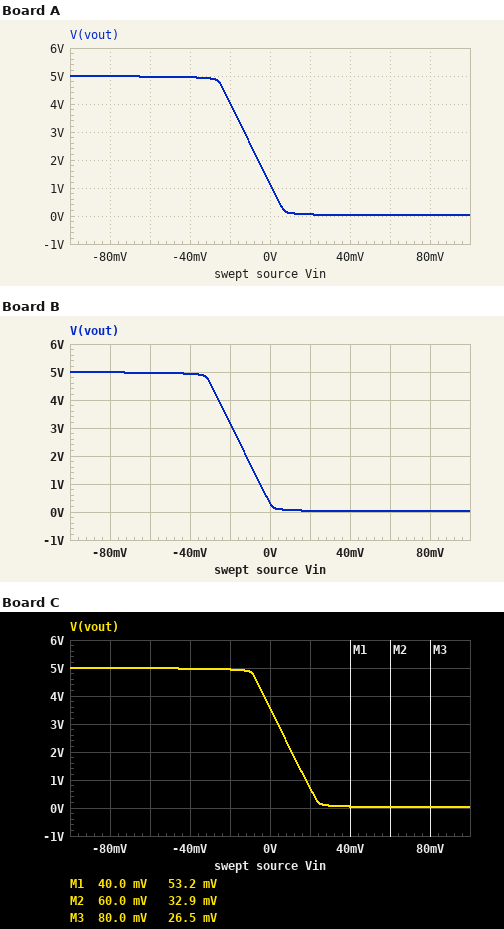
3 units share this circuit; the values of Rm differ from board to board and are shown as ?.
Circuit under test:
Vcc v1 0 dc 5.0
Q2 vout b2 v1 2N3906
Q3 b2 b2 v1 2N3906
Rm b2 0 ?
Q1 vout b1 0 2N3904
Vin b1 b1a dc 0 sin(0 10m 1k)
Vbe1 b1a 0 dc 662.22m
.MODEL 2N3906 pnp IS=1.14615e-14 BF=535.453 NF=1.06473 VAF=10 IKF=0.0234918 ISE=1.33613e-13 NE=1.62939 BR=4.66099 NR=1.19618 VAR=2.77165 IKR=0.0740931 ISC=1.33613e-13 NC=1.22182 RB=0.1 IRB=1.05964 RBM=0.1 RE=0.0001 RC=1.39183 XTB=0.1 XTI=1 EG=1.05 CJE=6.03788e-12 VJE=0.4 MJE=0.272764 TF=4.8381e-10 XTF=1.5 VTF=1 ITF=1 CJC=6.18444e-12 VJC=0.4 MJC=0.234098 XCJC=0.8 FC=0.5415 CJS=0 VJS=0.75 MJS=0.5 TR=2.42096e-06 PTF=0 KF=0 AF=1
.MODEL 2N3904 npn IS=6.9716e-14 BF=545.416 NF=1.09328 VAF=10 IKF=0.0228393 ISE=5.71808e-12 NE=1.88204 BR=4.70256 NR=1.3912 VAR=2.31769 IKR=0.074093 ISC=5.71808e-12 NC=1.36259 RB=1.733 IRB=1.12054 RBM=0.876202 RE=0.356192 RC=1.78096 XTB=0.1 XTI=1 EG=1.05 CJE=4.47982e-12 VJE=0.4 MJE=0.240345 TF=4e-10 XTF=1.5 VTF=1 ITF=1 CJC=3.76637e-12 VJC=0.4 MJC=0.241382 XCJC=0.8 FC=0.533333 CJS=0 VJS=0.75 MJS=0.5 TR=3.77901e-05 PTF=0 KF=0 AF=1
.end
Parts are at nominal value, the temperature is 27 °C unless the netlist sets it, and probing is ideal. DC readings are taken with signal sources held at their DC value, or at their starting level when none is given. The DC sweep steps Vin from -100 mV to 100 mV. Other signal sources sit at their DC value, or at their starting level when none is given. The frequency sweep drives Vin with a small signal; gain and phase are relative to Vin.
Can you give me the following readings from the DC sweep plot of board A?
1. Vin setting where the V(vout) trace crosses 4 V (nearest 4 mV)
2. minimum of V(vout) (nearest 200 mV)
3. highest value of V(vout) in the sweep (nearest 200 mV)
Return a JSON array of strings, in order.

["-20 mV", "0 V", "5.0 V"]
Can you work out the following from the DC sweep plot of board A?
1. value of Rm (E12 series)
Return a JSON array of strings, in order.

["8.2 kΩ"]
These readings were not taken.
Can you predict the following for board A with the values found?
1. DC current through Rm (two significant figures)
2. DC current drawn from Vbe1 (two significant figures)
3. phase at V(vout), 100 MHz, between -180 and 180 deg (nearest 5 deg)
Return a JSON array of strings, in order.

["530 µA", "6.5 µA", "100 deg"]
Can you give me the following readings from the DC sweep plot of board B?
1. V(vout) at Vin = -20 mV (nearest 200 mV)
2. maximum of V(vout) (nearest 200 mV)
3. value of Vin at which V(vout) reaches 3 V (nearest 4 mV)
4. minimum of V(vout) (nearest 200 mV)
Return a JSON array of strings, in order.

["3.2 V", "5.0 V", "-20 mV", "0 V"]
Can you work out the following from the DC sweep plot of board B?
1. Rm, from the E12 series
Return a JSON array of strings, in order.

["10 kΩ"]
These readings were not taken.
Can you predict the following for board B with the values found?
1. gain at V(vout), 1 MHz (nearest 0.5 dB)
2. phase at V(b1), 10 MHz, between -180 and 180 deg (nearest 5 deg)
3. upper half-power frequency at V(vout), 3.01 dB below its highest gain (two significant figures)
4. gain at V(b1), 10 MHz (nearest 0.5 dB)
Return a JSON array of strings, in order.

["39.0 dB", "0 deg", "1.2 MHz", "0 dB"]
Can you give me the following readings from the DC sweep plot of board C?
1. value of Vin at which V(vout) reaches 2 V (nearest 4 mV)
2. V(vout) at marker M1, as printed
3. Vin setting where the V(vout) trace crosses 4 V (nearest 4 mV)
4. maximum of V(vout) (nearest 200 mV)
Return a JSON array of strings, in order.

["12 mV", "53.2 mV", "-4 mV", "5.0 V"]
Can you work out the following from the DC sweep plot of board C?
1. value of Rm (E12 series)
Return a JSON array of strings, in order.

["4.7 kΩ"]
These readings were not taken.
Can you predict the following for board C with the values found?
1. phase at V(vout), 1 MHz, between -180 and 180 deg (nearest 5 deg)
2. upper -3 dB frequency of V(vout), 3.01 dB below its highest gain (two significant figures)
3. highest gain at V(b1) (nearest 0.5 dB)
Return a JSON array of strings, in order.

["160 deg", "2.7 MHz", "0 dB"]
